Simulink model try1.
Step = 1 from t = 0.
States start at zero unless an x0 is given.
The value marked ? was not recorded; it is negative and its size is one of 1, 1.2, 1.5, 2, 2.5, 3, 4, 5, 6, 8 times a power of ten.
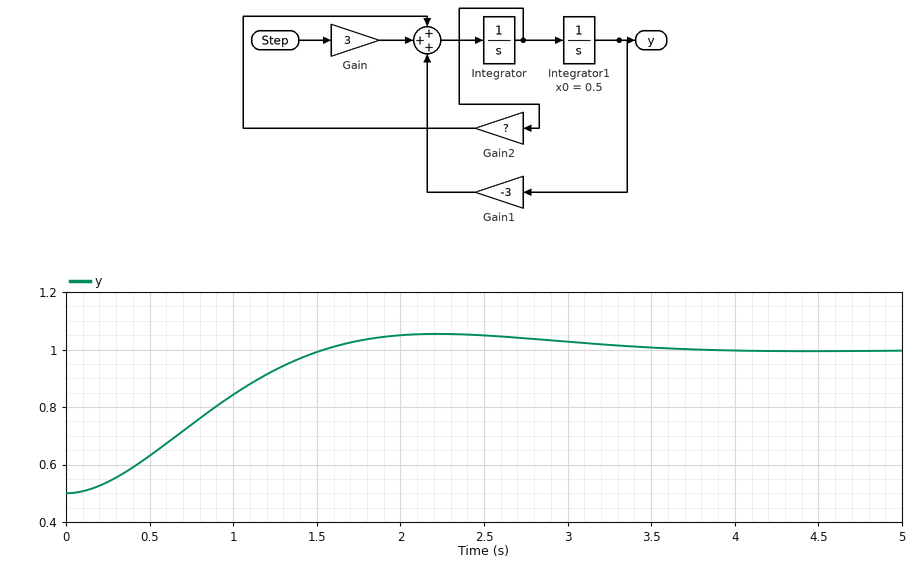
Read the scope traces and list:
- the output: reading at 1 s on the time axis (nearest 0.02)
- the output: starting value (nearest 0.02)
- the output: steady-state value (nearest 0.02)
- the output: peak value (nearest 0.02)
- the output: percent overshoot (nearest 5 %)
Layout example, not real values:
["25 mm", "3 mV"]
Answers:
["0.84", "0.50", "1.00", "1.06", "10 %"]
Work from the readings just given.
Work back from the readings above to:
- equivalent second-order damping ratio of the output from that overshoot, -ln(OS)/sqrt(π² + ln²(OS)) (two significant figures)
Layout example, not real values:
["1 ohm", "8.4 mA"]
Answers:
["0.59"]
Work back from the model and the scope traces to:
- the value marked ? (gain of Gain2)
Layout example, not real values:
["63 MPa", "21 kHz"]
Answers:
["-2"]
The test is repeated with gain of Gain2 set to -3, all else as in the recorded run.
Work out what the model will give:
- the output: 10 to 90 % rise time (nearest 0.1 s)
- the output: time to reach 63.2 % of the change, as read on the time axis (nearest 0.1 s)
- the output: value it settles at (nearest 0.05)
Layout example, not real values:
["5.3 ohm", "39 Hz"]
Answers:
["1.6 s", "1.1 s", "1.00"]
